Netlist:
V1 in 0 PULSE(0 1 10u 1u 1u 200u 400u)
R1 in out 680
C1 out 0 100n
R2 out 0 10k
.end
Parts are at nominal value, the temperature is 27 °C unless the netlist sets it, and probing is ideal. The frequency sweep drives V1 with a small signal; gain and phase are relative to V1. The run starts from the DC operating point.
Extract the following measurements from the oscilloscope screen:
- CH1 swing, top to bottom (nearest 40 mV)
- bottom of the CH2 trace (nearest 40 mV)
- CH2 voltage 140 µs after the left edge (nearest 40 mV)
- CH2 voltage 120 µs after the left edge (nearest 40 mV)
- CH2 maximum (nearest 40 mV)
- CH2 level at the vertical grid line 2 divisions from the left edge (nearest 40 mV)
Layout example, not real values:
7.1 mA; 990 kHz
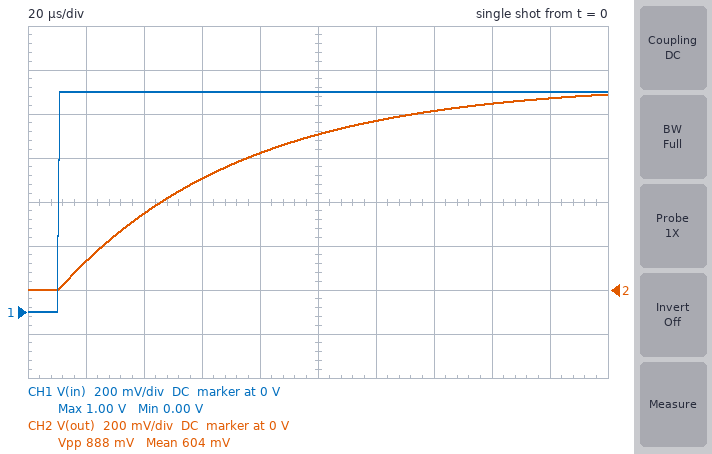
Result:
1.00 V; 0 V; 800 mV; 760 mV; 880 mV; 360 mV
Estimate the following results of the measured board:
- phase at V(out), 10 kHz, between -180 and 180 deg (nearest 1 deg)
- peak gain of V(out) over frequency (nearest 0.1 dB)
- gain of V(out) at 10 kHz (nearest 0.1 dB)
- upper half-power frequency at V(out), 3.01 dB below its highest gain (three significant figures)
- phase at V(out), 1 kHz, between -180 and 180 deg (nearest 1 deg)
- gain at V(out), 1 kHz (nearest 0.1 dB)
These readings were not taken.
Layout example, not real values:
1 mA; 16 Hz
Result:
-76 deg; -0.6 dB; -12.9 dB; 2.50 kHz; -22 deg; -1.2 dB
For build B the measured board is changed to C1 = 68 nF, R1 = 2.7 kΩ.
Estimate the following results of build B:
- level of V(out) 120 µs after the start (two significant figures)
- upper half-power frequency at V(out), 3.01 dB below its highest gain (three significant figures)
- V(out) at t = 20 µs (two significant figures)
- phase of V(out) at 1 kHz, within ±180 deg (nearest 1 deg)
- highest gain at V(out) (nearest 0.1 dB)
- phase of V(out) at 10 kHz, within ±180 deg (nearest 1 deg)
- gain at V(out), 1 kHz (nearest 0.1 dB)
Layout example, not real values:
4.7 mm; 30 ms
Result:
420 mV; 1.10 kHz; 50 mV; -42 deg; -2.1 dB; -84 deg; -4.7 dB
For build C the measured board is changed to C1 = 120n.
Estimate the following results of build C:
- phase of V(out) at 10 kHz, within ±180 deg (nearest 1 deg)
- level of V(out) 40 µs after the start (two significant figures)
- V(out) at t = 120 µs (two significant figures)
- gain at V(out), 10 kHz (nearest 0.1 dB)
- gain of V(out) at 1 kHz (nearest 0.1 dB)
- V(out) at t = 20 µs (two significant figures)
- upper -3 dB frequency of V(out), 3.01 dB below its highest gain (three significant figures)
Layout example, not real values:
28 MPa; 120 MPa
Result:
-78 deg; 300 mV; 710 mV; -14.4 dB; -1.5 dB; 110 mV; 2.08 kHz
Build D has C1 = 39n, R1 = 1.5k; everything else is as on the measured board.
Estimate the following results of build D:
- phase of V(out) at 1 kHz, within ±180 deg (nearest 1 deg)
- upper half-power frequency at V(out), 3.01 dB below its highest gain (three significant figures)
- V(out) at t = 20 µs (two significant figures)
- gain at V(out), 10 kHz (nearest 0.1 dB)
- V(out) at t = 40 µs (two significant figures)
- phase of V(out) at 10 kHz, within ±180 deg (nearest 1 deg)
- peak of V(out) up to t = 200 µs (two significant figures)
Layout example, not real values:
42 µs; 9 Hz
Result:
-18 deg; 3.13 kHz; 150 mV; -11.7 dB; 380 mV; -73 deg; 850 mV
